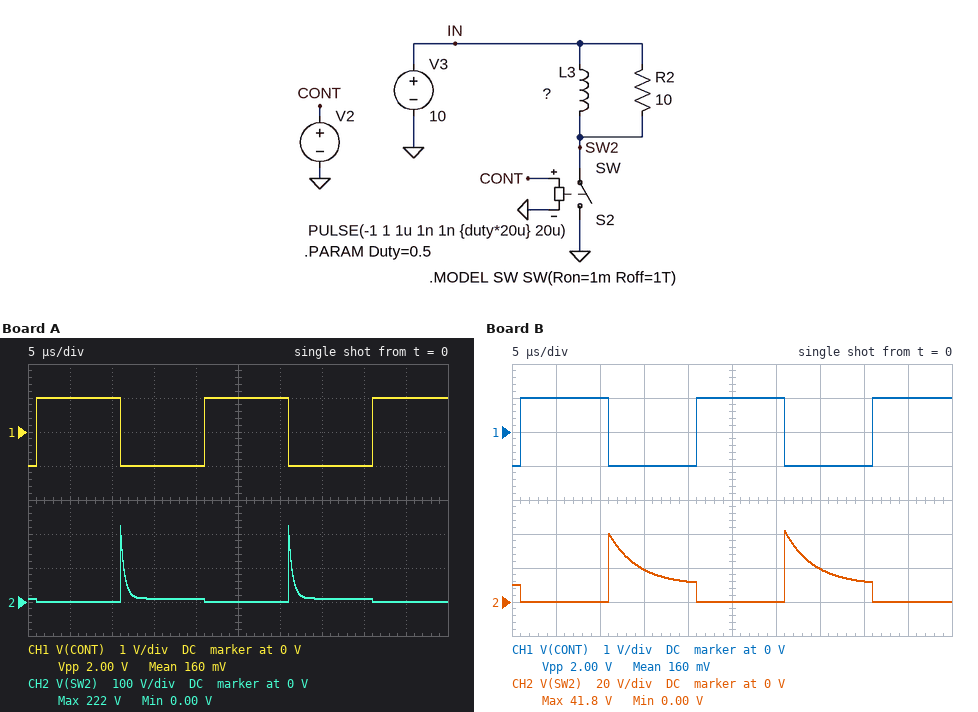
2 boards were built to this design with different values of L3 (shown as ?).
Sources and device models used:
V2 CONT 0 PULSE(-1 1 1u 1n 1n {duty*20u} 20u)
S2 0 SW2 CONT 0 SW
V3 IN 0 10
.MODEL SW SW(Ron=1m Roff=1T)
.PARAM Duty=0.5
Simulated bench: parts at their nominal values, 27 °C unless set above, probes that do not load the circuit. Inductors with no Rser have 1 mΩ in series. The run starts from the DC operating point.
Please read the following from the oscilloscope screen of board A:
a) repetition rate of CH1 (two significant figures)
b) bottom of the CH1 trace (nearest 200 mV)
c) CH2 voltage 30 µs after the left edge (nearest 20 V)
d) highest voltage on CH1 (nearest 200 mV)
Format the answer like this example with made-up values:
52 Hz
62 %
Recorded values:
50 kHz
-1.0 V
0 V
1.0 V
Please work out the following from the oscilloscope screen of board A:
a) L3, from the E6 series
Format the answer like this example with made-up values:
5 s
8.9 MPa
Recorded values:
4.7 µH
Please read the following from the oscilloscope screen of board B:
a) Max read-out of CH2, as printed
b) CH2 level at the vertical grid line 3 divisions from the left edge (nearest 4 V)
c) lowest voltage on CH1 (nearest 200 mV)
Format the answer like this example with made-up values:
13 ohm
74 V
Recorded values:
41.8 V
20 V
-1.0 V
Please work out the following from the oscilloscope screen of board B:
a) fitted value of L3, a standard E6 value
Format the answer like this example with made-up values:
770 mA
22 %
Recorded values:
33 µH
